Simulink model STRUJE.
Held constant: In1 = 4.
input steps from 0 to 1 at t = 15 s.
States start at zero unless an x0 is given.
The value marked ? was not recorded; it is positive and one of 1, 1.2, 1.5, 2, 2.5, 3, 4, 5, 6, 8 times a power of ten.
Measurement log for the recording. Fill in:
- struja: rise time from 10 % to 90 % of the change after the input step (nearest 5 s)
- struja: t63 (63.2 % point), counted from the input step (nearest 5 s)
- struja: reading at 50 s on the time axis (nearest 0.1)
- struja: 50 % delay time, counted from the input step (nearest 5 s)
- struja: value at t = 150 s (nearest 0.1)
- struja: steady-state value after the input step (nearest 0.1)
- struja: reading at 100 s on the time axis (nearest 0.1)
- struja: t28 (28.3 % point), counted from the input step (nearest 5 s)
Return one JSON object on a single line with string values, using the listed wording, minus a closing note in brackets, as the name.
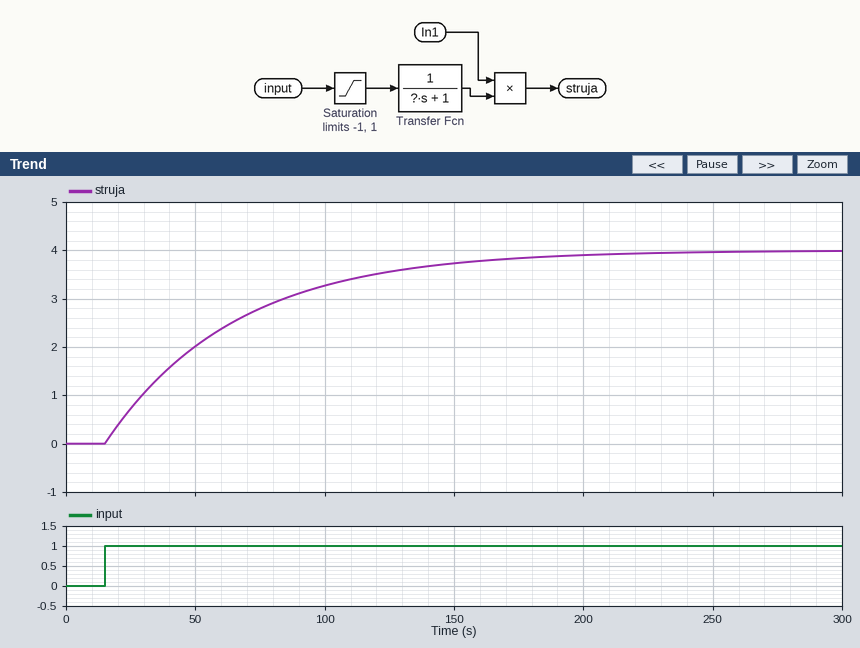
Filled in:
{"struja: rise time from 10 % to 90 % of the change after the input step": "110 s", "struja: t63 (63.2 % point), counted from the input step": "50 s", "struja: reading at 50 s on the time axis": "2.0", "struja: 50 % delay time, counted from the input step": "35 s", "struja: value at t = 150 s": "3.7", "struja: steady-state value after the input step": "4.0", "struja: reading at 100 s on the time axis": "3.3", "struja: t28 (28.3 % point), counted from the input step": "15 s"}
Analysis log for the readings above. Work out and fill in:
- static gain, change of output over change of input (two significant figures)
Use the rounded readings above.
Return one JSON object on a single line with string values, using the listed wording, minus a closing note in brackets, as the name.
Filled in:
{"static gain, change of output over change of input": "4.0"}
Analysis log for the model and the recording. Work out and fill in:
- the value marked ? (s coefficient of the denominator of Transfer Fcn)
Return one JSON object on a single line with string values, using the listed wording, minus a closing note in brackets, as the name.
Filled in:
{"the value marked ?": "50"}
